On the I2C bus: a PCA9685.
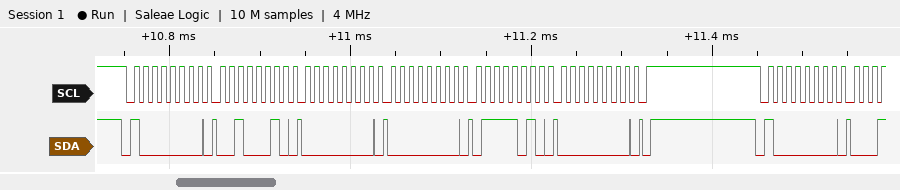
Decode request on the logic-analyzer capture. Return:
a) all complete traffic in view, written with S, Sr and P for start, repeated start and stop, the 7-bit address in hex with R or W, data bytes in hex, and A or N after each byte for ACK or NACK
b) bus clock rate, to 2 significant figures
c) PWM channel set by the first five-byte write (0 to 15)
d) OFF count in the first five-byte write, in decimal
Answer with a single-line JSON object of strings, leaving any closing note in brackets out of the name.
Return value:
{"all complete traffic in view, written with S, Sr and P for start, repeated start and stop, the 7-bit address in hex with R or W, data bytes in hex, and A or N after each byte for ACK or NACK": "S 40W A 22 A 00 A 00 A 7A A 00 A P S 40W A", "bus clock rate, to 2 significant figures": "100 kHz", "PWM channel set by the first five-byte write": "7", "OFF count in the first five-byte write, in decimal": "122"}
